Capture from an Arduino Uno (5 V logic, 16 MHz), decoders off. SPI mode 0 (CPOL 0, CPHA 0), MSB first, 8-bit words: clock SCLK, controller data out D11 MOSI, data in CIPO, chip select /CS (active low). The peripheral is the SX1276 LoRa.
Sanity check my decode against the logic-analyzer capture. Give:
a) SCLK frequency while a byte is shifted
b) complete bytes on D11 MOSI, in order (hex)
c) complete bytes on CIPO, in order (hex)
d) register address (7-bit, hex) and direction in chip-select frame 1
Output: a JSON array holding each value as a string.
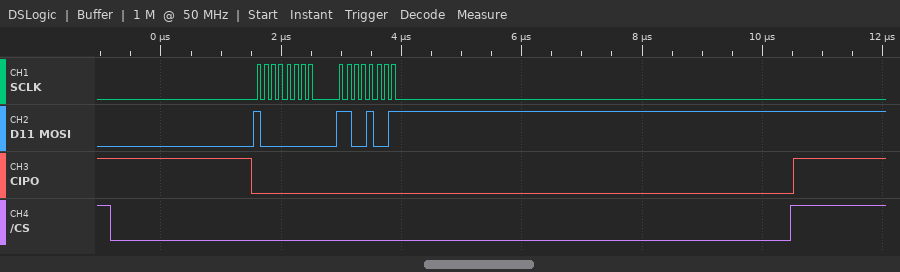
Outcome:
["8 MHz", "80 C9", "00 00", "0x00 write"]
